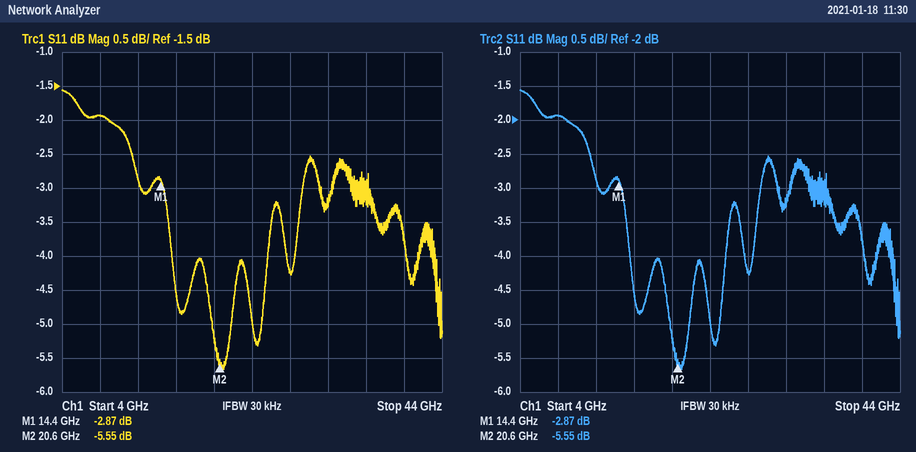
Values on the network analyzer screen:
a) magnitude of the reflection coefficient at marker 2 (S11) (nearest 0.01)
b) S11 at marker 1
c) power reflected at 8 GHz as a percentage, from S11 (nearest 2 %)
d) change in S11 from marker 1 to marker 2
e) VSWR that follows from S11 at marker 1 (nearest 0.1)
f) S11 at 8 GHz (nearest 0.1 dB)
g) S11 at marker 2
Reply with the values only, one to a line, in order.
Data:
0.53
-2.87 dB
64 %
-2.68 dB
6.1
-1.9 dB
-5.55 dB
